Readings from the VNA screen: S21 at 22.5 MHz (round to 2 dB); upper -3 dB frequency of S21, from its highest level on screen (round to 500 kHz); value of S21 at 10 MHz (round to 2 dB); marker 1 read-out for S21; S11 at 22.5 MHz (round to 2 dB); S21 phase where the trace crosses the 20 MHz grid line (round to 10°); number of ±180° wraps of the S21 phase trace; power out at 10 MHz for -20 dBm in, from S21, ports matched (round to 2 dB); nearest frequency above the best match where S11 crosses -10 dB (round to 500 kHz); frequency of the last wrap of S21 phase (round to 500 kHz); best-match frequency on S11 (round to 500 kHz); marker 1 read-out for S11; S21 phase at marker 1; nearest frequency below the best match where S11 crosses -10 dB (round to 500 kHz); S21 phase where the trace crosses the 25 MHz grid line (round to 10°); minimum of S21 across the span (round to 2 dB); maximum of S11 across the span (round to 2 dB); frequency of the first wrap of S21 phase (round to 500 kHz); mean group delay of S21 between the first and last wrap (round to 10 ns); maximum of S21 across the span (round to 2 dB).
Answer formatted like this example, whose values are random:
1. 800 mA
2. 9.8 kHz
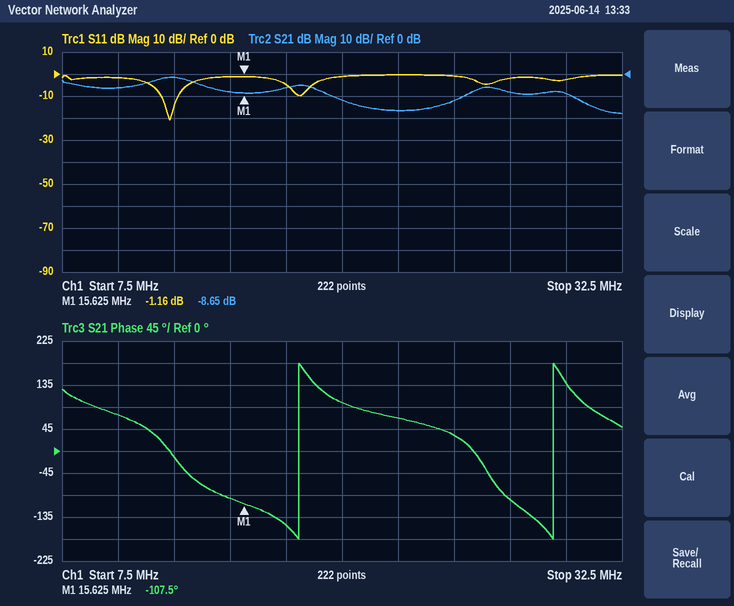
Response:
1. -16 dB
2. 13.5 MHz
3. -6 dB
4. -8.65 dB
5. 0 dB
6. 100°
7. 2
8. -26 dBm
9. 12.5 MHz
10. 29.5 MHz
11. 12.5 MHz
12. -1.16 dB
13. -107.5°
14. 12.0 MHz
15. 30°
16. -18 dB
17. 0 dB
18. 18.0 MHz
19. 90 ns
20. -2 dB
